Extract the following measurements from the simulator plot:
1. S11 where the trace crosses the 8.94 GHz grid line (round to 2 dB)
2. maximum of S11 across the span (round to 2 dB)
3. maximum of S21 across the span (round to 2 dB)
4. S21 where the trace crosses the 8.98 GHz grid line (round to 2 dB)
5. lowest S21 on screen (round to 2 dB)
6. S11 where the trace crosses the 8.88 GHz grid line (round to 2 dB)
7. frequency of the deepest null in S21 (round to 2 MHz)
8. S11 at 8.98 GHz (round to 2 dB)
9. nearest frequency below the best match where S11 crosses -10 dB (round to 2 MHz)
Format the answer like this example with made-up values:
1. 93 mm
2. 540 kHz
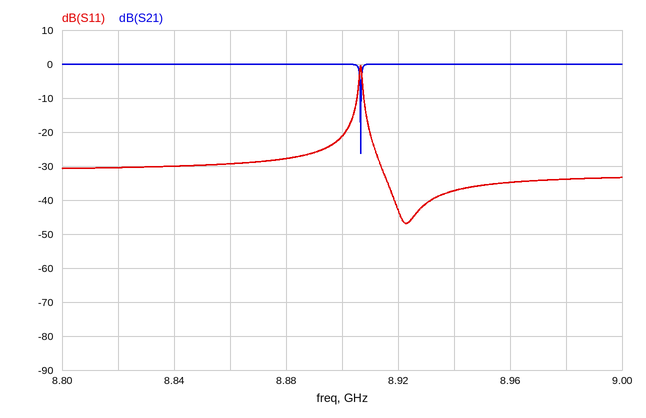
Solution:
1. -38 dB
2. 0 dB
3. 0 dB
4. 0 dB
5. -26 dB
6. -28 dB
7. 8.906 GHz
8. -34 dB
9. 8.908 GHz
